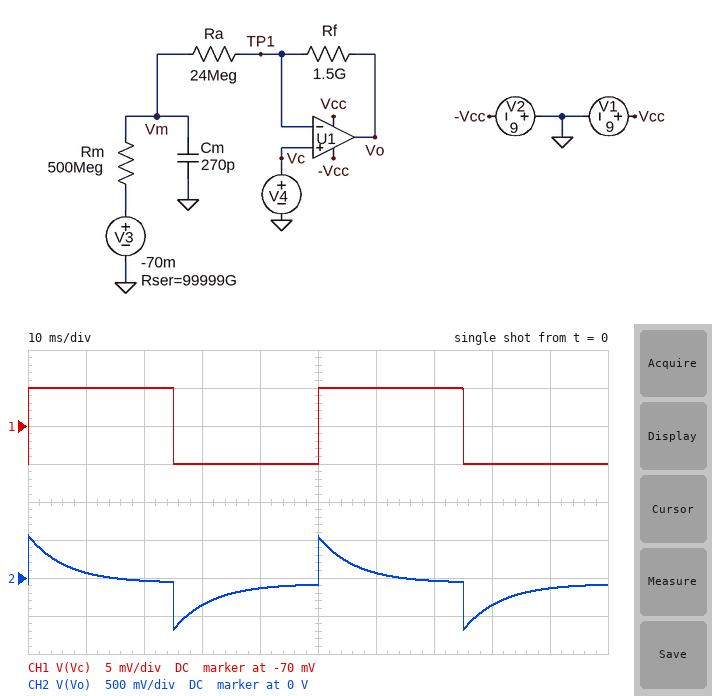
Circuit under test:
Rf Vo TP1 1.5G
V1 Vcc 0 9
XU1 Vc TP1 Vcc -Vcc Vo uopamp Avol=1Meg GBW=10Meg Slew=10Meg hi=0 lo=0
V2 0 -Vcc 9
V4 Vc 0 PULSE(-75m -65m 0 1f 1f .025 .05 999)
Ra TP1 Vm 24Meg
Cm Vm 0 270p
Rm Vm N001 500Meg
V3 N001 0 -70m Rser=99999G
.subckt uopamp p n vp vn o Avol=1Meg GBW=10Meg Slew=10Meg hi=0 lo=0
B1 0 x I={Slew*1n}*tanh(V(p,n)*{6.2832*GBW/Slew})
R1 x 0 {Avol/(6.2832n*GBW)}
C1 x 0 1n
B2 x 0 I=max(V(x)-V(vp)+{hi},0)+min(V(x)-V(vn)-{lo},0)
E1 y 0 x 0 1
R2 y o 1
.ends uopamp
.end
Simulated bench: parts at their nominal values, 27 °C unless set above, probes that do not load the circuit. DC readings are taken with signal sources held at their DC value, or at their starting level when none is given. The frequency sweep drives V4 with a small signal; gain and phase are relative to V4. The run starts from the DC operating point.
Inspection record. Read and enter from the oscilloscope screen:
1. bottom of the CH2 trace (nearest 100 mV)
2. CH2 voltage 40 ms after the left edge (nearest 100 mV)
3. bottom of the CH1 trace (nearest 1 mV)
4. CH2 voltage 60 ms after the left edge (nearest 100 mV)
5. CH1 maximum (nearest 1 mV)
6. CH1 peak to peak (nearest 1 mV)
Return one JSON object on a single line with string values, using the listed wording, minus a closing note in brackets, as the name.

{"bottom of the CH2 trace": "-700 mV", "CH2 voltage 40 ms after the left edge": "-100 mV", "bottom of the CH1 trace": "-75 mV", "CH2 voltage 60 ms after the left edge": "100 mV", "CH1 maximum": "-65 mV", "CH1 peak to peak": "10 mV"}
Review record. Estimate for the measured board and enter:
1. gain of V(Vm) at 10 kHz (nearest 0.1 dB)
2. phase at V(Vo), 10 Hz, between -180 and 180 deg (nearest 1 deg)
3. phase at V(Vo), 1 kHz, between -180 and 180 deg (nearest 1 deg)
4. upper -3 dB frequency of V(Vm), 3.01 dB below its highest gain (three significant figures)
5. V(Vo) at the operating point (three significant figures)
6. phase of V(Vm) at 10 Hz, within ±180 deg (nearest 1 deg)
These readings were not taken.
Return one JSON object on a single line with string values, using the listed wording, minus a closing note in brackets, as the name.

{"gain of V(Vm) at 10 kHz": "-52.2 dB", "phase at V(Vo), 10 Hz, between -180 and 180 deg": "66 deg", "phase at V(Vo), 1 kHz, between -180 and 180 deg": "1 deg", "upper -3 dB frequency of V(Vm), 3.01 dB below its highest gain": "24.6 Hz", "V(Vo) at the operating point": "-75.0 mV", "phase of V(Vm) at 10 Hz, within ±180 deg": "-22 deg"}
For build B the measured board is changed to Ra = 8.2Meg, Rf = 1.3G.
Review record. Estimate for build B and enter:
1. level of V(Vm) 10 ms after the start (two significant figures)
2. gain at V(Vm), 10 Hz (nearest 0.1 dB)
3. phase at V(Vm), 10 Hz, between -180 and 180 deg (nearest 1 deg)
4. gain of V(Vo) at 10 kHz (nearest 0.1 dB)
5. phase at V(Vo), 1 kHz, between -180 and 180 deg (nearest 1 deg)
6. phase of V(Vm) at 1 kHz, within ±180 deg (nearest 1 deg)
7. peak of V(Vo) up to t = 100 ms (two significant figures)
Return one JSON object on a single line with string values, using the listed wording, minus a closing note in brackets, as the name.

{"level of V(Vm) 10 ms after the start": "-65 mV", "gain at V(Vm), 10 Hz": "-0.1 dB", "phase at V(Vm), 10 Hz, between -180 and 180 deg": "-8 deg", "gain of V(Vo) at 10 kHz": "44.0 dB", "phase at V(Vo), 1 kHz, between -180 and 180 deg": "3 deg", "phase of V(Vm) at 1 kHz, within ±180 deg": "-87 deg", "peak of V(Vo) up to t = 100 ms": "1.5 V"}
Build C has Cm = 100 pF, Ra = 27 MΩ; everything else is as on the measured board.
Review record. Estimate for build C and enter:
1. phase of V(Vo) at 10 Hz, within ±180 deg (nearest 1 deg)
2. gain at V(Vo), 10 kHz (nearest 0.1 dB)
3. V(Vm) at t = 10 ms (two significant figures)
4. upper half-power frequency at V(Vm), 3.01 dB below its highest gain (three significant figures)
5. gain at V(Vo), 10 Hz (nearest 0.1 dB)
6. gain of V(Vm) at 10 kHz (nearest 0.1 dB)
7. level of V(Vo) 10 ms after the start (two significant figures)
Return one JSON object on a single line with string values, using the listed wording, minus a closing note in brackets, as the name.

{"phase of V(Vo) at 10 Hz, within ±180 deg": "74 deg", "gain at V(Vo), 10 kHz": "35.0 dB", "V(Vm) at t = 10 ms": "-65 mV", "upper half-power frequency at V(Vm), 3.01 dB below its highest gain": "59.0 Hz", "gain at V(Vo), 10 Hz": "19.6 dB", "gain of V(Vm) at 10 kHz": "-44.6 dB", "level of V(Vo) 10 ms after the start": "-51 mV"}
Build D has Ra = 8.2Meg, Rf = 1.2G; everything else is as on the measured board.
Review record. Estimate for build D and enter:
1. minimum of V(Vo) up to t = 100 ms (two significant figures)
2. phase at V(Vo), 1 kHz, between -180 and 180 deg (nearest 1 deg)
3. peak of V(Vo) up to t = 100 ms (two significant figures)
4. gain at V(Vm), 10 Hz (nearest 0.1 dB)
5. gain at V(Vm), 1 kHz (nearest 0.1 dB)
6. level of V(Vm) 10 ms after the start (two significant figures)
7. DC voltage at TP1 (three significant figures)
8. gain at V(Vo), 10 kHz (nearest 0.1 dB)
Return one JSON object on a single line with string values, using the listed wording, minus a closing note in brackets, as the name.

{"minimum of V(Vo) up to t = 100 ms": "-1.5 V", "phase at V(Vo), 1 kHz, between -180 and 180 deg": "3 deg", "peak of V(Vo) up to t = 100 ms": "1.4 V", "gain at V(Vm), 10 Hz": "-0.1 dB", "gain at V(Vm), 1 kHz": "-22.9 dB", "level of V(Vm) 10 ms after the start": "-65 mV", "DC voltage at TP1": "-75.0 mV", "gain at V(Vo), 10 kHz": "43.3 dB"}
